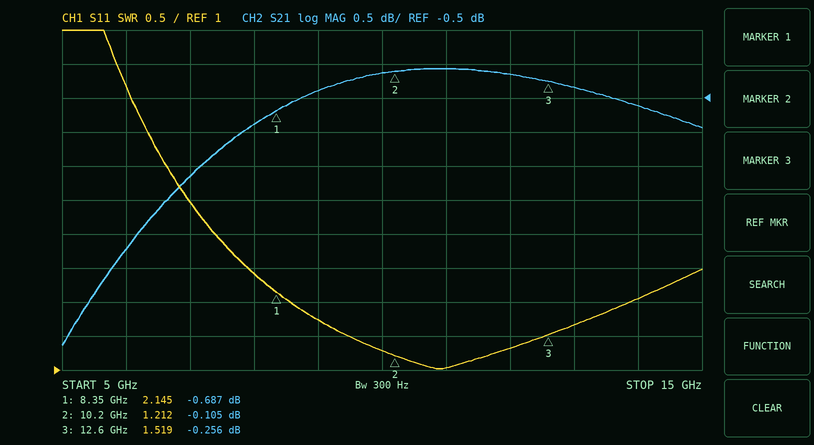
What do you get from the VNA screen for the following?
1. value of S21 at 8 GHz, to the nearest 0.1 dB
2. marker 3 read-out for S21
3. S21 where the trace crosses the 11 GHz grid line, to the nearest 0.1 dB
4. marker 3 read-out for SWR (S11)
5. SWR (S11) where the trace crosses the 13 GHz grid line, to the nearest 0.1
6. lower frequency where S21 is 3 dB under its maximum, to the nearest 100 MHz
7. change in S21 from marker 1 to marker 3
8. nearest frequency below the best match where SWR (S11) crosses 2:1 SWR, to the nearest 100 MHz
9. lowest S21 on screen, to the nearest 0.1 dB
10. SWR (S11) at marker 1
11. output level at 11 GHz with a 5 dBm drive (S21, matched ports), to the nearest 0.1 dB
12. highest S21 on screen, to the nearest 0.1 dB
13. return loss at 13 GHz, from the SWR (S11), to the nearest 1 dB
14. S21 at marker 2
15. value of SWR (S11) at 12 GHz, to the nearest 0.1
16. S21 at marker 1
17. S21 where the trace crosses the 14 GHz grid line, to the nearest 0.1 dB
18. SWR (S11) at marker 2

-0.9 dB
-0.256 dB
-0.1 dB
1.519
1.7
5.7 GHz
0.431 dB
8.6 GHz
-4.1 dB
2.145
4.9 dBm
-0.1 dB
12 dB
-0.105 dB
1.3
-0.687 dB
-0.6 dB
1.212
